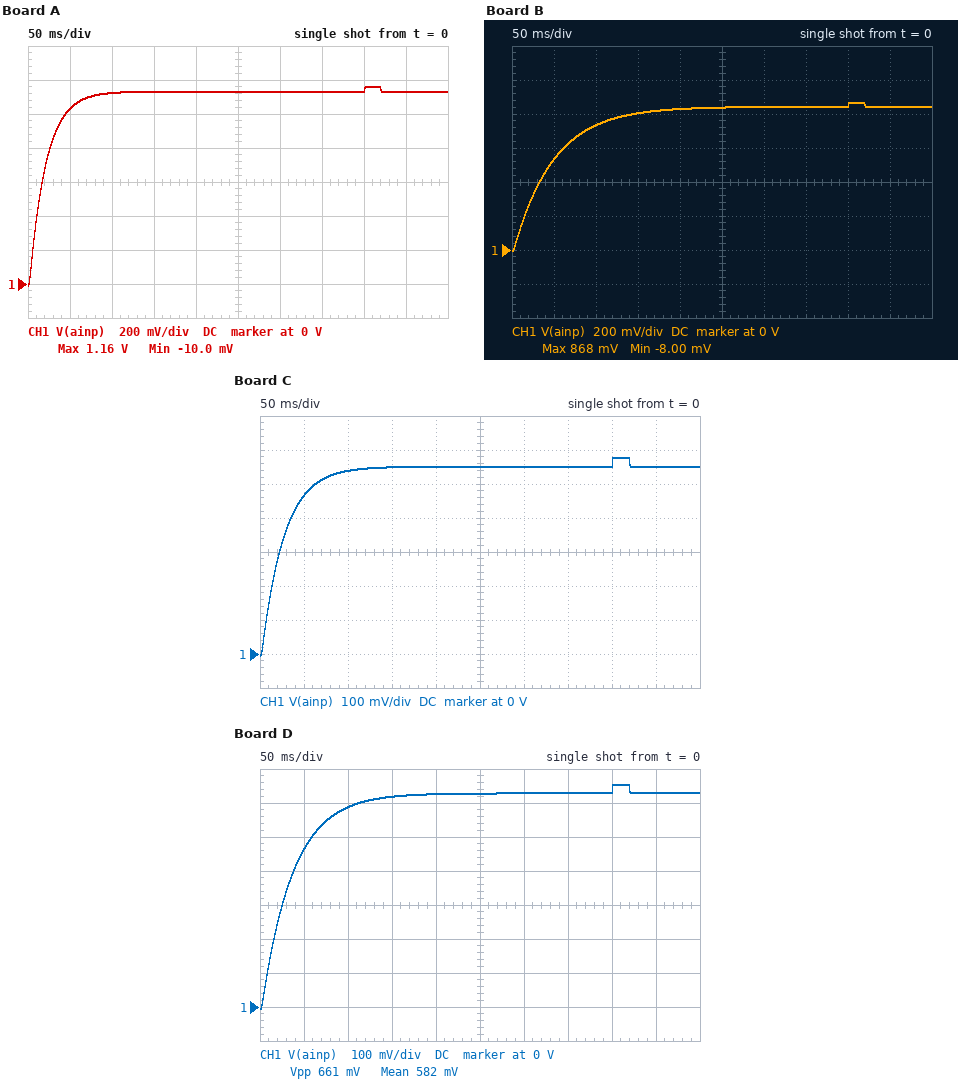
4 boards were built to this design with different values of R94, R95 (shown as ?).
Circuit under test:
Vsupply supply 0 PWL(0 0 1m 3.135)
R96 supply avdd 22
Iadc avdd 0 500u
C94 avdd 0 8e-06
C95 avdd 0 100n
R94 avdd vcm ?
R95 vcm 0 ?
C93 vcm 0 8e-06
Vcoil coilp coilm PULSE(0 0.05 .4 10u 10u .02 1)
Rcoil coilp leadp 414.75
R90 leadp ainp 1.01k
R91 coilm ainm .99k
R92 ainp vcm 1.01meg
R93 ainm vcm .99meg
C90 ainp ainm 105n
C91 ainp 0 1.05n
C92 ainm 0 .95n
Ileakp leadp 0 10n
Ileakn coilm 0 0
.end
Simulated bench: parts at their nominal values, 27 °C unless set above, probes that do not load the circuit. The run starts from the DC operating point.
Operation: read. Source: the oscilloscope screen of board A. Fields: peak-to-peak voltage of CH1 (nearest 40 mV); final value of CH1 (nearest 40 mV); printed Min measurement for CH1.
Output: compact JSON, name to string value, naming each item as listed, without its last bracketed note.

{"peak-to-peak voltage of CH1": "1.16 V", "final value of CH1": "1.12 V", "printed Min measurement for CH1": "-10.0 mV"}
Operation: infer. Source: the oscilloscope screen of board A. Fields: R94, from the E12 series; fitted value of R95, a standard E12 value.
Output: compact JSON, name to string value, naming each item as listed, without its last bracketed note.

{"R94, from the E12 series": "6.8 kΩ", "fitted value of R95, a standard E12 value": "3.9 kΩ"}
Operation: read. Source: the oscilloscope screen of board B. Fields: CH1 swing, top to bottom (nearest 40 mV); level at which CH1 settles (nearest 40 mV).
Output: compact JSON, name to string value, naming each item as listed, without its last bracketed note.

{"CH1 swing, top to bottom": "880 mV", "level at which CH1 settles": "840 mV"}
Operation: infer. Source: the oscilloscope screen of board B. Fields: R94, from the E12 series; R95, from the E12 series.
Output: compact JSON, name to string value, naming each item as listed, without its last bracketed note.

{"R94, from the E12 series": "22 kΩ", "R95, from the E12 series": "8.2 kΩ"}
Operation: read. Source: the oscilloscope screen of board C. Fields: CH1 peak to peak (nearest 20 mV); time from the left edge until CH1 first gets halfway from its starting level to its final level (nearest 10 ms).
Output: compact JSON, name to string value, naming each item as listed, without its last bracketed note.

{"CH1 peak to peak": "580 mV", "time from the left edge until CH1 first gets halfway from its starting level to its final level": "20 ms"}
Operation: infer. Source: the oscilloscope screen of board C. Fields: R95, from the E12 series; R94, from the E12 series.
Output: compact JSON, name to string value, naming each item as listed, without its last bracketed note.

{"R95, from the E12 series": "3.9 kΩ", "R94, from the E12 series": "18 kΩ"}
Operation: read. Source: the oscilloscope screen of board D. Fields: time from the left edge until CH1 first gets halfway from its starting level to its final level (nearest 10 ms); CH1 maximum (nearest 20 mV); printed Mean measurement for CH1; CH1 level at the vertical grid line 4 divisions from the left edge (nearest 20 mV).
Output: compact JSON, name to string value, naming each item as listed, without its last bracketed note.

{"time from the left edge until CH1 first gets halfway from its starting level to its final level": "30 ms", "CH1 maximum": "660 mV", "printed Mean measurement for CH1": "582 mV", "CH1 level at the vertical grid line 4 divisions from the left edge": "620 mV"}
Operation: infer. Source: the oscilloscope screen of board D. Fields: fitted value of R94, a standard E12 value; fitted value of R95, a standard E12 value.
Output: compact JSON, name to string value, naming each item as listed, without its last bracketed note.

{"fitted value of R94, a standard E12 value": "22 kΩ", "fitted value of R95, a standard E12 value": "5.6 kΩ"}
